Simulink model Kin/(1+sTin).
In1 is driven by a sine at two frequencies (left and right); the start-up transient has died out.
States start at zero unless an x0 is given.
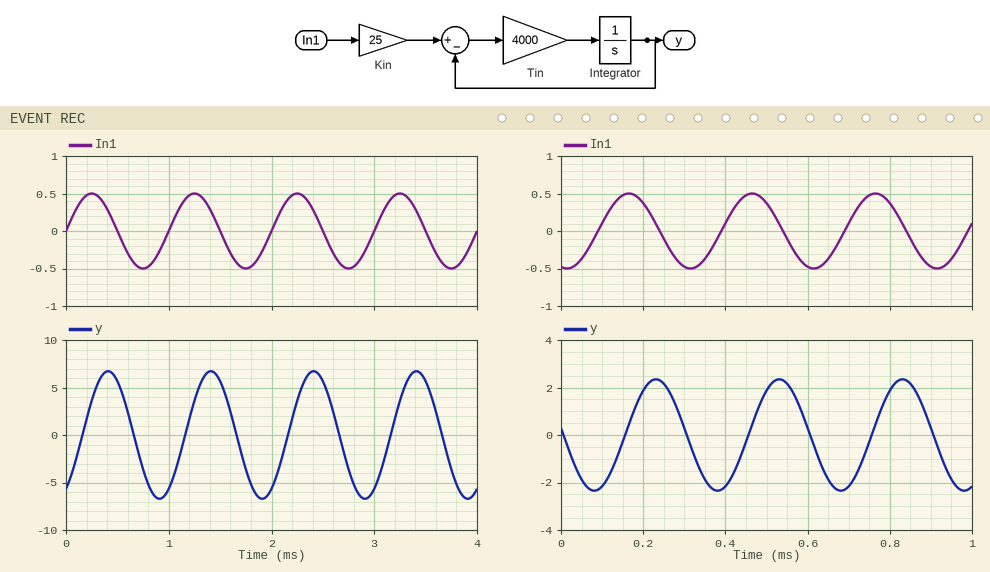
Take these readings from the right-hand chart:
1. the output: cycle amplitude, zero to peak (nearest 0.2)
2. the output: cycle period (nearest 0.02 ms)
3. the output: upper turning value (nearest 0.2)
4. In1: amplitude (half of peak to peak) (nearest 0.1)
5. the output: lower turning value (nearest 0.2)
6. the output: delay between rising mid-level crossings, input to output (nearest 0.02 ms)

2.4
0.30 ms
2.4
0.5
-2.4
0.06 ms
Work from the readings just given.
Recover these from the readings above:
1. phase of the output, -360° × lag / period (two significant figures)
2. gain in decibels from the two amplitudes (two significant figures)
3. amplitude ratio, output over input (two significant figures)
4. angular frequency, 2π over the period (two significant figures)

-72°
14 dB
4.8
21 rad/ms
